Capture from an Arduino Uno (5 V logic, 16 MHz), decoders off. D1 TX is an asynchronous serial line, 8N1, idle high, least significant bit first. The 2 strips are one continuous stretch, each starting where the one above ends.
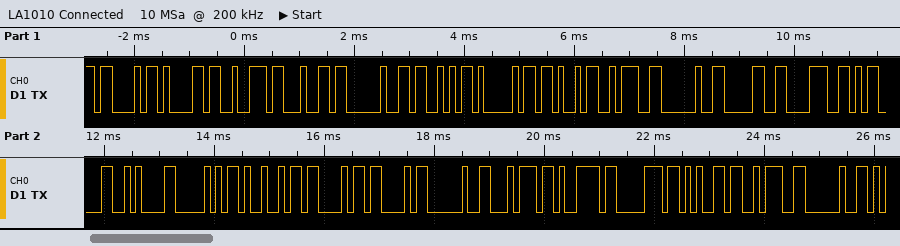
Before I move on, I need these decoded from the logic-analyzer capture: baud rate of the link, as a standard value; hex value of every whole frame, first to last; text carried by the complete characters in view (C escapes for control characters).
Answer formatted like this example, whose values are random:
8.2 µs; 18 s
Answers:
9600 baud; 43 61 72 64 20 53 41 4B 3A 20 30 38 0D 0A 50 49 43 43 20 74 79 70 65 3A 20; "Card SAK: 08\r\nPICC type: "
